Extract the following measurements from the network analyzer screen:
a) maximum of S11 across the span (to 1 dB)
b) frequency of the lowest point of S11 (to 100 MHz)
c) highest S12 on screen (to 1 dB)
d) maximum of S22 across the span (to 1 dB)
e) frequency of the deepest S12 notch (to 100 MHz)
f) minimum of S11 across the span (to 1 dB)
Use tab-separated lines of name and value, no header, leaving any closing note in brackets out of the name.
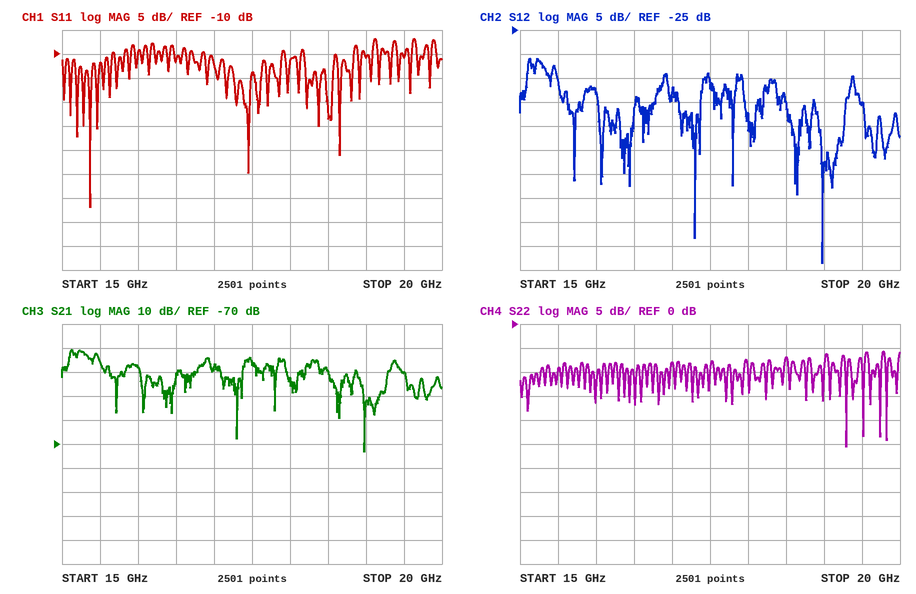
maximum of S11 across the span	-7 dB
frequency of the lowest point of S11	15.4 GHz
highest S12 on screen	-31 dB
maximum of S22 across the span	-6 dB
frequency of the deepest S12 notch	19.0 GHz
minimum of S11 across the span	-42 dB
